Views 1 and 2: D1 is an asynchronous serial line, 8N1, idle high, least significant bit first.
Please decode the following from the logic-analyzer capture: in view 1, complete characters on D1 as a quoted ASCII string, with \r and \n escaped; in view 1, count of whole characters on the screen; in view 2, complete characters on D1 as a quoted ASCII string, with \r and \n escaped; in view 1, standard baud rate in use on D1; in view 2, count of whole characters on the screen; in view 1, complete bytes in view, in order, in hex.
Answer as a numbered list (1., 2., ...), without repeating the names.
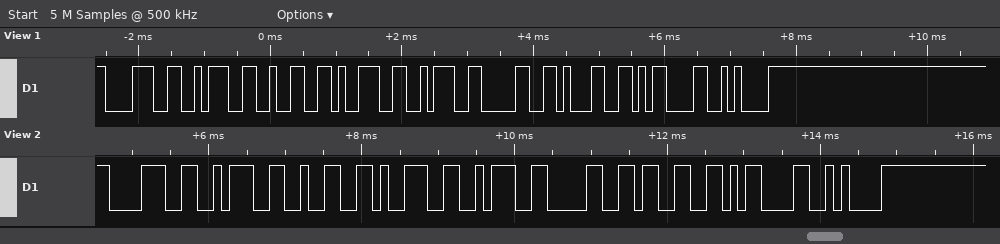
1. "8:29:01\r\n"
2. 9
3. "8:29:03\r\n"
4. 9600 baud
5. 9
6. 38 3A 32 39 3A 30 31 0D 0A
